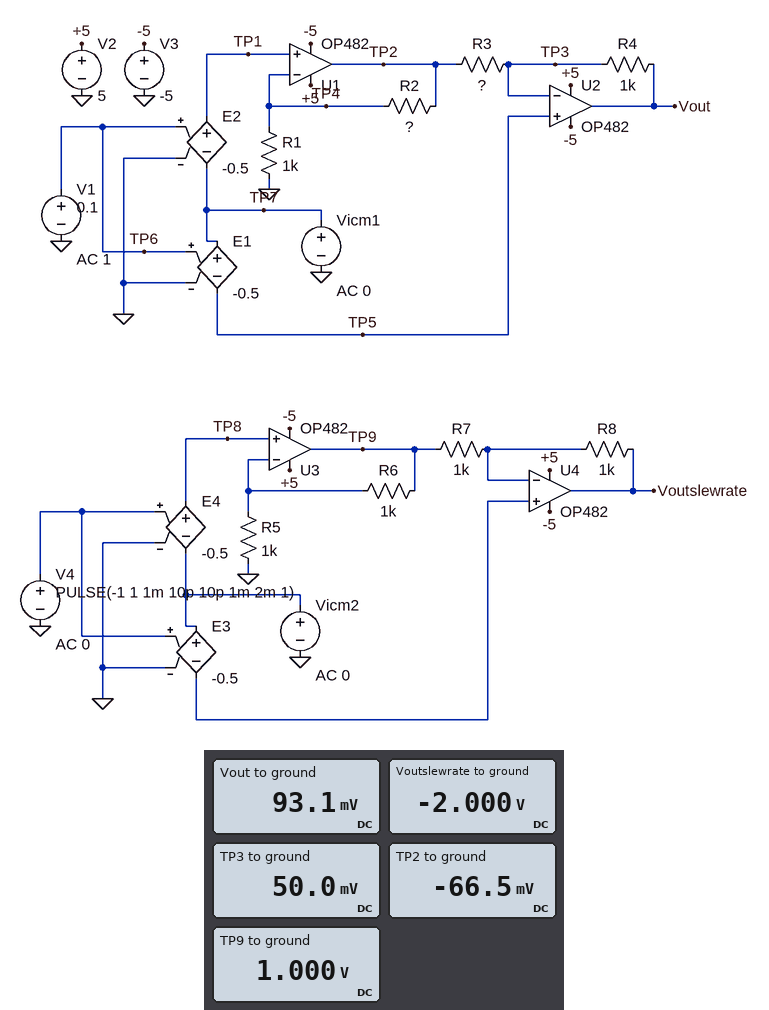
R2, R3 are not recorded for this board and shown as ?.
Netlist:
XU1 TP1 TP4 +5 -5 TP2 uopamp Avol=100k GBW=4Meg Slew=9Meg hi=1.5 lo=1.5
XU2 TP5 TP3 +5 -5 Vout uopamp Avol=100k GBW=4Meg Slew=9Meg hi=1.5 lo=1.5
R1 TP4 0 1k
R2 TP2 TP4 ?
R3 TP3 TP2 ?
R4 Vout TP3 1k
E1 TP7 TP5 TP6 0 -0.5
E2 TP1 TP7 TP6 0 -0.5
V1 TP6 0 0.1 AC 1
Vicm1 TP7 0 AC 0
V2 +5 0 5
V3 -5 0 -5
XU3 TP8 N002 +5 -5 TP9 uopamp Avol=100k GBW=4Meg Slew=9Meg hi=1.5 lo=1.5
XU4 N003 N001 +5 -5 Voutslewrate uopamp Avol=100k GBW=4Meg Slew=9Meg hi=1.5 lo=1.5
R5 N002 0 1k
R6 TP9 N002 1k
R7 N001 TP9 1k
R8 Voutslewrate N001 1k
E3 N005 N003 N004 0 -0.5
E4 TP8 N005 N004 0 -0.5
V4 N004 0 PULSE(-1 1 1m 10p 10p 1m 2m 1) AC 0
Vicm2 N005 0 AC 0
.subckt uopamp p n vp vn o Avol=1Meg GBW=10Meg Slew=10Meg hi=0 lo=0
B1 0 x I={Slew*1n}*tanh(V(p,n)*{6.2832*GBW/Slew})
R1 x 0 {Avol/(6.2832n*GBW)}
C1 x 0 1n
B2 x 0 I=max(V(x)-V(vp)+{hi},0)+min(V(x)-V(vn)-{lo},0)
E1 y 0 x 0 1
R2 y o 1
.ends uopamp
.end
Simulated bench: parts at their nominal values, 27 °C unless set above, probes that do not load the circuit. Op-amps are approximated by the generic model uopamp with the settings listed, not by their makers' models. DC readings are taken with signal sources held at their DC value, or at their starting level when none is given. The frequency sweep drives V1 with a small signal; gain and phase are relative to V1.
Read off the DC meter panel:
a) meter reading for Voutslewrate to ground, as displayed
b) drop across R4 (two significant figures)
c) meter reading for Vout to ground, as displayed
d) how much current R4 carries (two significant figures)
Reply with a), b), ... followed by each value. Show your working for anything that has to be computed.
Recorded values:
a) -2.000 V
b) 93.1 mV - 50 mV = 43 mV
c) 93.1 mV
d) (93.1 mV - 50 mV) / 1 kΩ = 43 µA
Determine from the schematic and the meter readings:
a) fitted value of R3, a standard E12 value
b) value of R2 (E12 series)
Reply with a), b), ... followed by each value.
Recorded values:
a) 2.7 kΩ
b) 330 Ω
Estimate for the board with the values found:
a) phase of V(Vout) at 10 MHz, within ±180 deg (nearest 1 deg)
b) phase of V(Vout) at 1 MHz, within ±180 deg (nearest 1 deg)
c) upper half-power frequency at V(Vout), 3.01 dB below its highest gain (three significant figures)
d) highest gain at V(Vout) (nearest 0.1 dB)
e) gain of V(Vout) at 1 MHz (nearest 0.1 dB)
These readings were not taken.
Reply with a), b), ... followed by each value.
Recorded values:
a) -79 deg
b) -24 deg
c) 2.35 MHz
d) -0.6 dB
e) -1.3 dB
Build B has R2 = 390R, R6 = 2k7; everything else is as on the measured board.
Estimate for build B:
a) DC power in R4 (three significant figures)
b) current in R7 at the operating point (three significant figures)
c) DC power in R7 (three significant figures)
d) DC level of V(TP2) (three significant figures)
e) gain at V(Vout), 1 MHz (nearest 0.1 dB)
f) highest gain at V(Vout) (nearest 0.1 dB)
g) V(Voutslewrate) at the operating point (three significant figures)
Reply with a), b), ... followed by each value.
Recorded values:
a) 1.96 µW
b) 2.35 mA
c) 5.52 mW
d) -69.5 mV
e) -1.2 dB
f) -0.5 dB
g) -2.85 V
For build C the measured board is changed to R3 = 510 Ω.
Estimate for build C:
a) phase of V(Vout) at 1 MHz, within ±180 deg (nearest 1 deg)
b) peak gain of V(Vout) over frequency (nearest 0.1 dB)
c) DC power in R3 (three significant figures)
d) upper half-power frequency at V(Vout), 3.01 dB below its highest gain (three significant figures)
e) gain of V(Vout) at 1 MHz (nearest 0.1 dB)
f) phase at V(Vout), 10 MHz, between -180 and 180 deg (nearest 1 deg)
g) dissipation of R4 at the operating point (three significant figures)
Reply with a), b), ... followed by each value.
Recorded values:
a) -45 deg
b) 8.9 dB
c) 26.6 µW
d) 1.21 MHz
e) 6.7 dB
f) -95 deg
g) 52.2 µW
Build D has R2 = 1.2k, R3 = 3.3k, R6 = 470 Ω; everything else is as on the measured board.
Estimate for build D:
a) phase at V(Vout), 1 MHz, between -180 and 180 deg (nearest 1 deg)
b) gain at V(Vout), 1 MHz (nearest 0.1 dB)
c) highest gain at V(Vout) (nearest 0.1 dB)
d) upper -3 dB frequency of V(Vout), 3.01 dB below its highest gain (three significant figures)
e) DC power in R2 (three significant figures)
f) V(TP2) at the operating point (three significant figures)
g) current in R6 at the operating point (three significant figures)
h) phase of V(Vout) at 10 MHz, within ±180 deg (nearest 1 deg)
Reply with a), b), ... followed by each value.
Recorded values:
a) -27 deg
b) -1.2 dB
c) -0.1 dB
d) 1.94 MHz
e) 3.00 µW
f) -110 mV
g) 500 µA
h) -78 deg
